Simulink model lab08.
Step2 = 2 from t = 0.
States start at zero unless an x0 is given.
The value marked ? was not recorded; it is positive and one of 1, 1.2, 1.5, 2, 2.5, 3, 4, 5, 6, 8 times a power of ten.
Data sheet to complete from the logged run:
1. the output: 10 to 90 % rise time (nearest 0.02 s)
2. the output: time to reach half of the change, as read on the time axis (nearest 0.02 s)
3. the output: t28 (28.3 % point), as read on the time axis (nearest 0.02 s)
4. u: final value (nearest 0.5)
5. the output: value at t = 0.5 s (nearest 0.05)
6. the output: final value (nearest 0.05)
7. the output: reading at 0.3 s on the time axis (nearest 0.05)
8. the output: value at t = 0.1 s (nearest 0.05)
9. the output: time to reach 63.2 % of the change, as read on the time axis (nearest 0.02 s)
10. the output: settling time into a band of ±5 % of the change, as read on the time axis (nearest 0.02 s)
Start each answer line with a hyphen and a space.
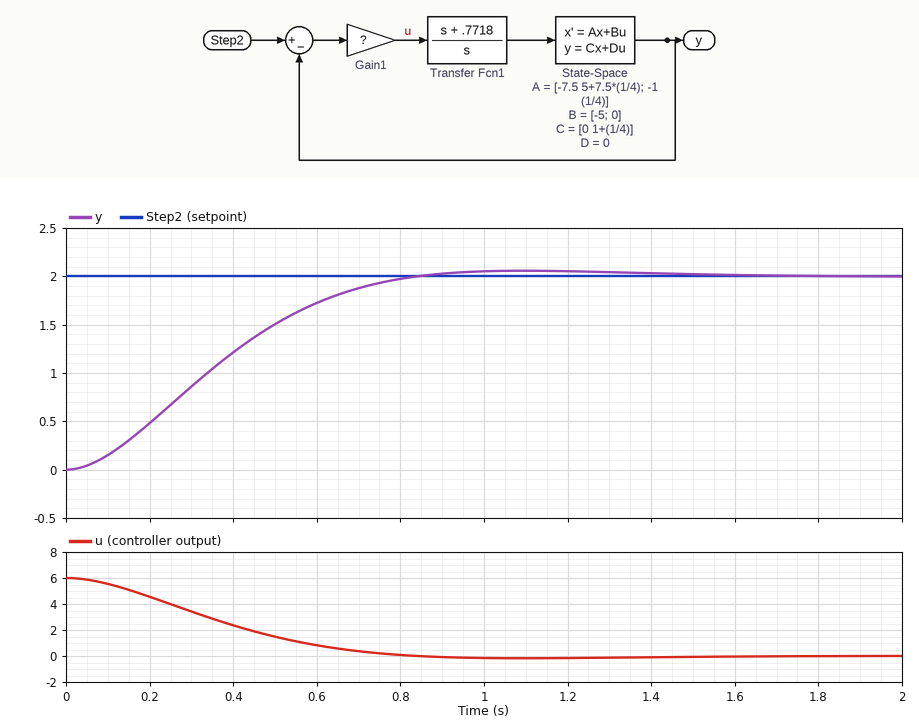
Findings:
- 0.52 s
- 0.34 s
- 0.22 s
- 0.0
- 1.50
- 2.00
- 0.85
- 0.15
- 0.42 s
- 0.72 s
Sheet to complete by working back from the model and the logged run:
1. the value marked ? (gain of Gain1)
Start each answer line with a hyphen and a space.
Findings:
- 3
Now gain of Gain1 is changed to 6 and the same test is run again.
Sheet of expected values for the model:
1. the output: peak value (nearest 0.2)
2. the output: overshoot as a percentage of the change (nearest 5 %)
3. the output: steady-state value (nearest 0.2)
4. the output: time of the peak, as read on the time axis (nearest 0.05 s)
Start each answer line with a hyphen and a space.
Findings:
- 2.2
- 15 %
- 2.0
- 0.60 s
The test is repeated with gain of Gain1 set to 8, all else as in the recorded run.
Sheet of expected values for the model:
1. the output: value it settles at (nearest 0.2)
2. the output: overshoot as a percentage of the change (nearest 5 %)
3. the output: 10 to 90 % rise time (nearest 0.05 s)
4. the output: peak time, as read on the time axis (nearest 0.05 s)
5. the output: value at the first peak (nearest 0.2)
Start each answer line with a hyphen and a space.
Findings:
- 2.0
- 20 %
- 0.20 s
- 0.50 s
- 2.4
